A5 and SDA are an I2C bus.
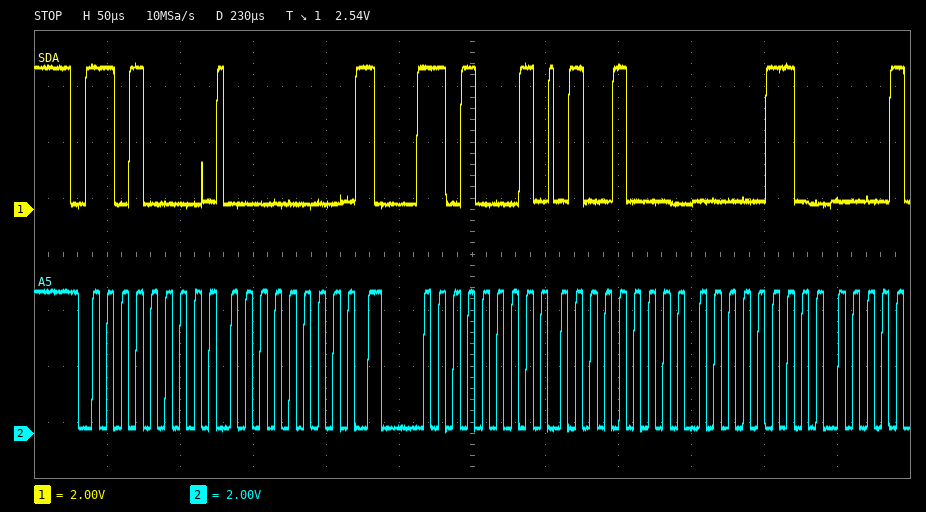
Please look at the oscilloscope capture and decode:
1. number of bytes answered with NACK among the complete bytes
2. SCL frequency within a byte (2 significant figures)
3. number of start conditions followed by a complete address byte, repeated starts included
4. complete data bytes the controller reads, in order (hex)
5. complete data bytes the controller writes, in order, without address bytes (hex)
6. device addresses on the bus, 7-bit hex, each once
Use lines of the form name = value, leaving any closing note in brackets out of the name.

number of bytes answered with NACK among the complete bytes = 0
SCL frequency within a byte = 100 kHz
number of start conditions followed by a complete address byte, repeated starts included = 2
complete data bytes the controller reads, in order = 48 06
complete data bytes the controller writes, in order, without address bytes = 00
device addresses on the bus, 7-bit hex, each once = 0x68
